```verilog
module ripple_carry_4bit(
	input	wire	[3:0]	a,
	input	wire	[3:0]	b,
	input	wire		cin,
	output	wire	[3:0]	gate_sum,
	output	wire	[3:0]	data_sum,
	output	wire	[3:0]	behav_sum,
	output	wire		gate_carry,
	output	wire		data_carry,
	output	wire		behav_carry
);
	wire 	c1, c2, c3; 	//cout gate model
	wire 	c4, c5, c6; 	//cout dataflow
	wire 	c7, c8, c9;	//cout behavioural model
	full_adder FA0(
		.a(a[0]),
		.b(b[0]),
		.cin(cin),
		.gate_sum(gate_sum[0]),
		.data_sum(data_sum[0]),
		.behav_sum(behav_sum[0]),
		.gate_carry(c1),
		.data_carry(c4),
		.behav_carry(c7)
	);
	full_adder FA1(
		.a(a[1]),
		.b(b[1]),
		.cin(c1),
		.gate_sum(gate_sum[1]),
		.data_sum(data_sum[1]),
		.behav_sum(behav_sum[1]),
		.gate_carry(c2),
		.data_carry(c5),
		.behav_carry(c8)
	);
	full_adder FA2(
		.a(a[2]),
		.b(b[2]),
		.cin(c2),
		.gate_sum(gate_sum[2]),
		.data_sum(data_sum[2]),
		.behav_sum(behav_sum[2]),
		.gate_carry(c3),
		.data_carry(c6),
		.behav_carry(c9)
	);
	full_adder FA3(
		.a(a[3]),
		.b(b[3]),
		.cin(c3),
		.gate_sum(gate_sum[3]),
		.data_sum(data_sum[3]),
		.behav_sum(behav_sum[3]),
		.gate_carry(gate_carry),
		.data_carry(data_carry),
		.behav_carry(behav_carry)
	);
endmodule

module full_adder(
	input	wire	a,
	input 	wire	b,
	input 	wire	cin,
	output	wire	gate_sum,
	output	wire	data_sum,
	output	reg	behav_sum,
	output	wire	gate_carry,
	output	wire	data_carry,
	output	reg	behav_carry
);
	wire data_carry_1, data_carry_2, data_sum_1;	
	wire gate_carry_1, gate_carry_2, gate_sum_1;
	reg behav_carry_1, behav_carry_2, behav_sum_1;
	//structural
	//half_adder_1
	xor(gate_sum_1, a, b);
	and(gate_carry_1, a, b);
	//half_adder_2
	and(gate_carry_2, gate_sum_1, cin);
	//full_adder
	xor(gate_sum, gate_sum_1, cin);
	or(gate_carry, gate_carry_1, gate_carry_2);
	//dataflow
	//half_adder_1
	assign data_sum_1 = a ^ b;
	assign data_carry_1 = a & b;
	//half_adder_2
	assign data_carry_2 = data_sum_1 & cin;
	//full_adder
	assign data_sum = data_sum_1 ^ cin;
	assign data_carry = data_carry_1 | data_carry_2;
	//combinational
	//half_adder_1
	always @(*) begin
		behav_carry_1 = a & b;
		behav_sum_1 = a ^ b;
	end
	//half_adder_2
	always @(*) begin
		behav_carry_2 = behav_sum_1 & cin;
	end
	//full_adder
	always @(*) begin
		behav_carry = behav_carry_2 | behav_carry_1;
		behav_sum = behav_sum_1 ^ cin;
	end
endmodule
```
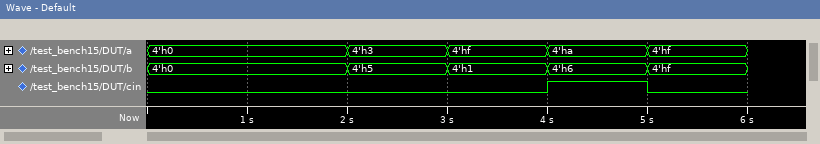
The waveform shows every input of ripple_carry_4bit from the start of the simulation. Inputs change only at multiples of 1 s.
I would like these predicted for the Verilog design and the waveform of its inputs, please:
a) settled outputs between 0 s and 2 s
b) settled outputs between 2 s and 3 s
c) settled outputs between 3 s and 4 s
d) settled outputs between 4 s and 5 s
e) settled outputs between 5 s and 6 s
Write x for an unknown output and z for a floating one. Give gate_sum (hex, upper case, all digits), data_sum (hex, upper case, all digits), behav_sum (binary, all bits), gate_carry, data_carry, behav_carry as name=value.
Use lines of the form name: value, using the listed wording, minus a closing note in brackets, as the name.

settled outputs between 0 s and 2 s: gate_sum=0, data_sum=0, behav_sum=0000, gate_carry=0, data_carry=0, behav_carry=0
settled outputs between 2 s and 3 s: gate_sum=8, data_sum=8, behav_sum=1000, gate_carry=0, data_carry=0, behav_carry=0
settled outputs between 3 s and 4 s: gate_sum=0, data_sum=0, behav_sum=0000, gate_carry=1, data_carry=1, behav_carry=1
settled outputs between 4 s and 5 s: gate_sum=1, data_sum=1, behav_sum=0001, gate_carry=1, data_carry=1, behav_carry=1
settled outputs between 5 s and 6 s: gate_sum=E, data_sum=E, behav_sum=1110, gate_carry=1, data_carry=1, behav_carry=1
